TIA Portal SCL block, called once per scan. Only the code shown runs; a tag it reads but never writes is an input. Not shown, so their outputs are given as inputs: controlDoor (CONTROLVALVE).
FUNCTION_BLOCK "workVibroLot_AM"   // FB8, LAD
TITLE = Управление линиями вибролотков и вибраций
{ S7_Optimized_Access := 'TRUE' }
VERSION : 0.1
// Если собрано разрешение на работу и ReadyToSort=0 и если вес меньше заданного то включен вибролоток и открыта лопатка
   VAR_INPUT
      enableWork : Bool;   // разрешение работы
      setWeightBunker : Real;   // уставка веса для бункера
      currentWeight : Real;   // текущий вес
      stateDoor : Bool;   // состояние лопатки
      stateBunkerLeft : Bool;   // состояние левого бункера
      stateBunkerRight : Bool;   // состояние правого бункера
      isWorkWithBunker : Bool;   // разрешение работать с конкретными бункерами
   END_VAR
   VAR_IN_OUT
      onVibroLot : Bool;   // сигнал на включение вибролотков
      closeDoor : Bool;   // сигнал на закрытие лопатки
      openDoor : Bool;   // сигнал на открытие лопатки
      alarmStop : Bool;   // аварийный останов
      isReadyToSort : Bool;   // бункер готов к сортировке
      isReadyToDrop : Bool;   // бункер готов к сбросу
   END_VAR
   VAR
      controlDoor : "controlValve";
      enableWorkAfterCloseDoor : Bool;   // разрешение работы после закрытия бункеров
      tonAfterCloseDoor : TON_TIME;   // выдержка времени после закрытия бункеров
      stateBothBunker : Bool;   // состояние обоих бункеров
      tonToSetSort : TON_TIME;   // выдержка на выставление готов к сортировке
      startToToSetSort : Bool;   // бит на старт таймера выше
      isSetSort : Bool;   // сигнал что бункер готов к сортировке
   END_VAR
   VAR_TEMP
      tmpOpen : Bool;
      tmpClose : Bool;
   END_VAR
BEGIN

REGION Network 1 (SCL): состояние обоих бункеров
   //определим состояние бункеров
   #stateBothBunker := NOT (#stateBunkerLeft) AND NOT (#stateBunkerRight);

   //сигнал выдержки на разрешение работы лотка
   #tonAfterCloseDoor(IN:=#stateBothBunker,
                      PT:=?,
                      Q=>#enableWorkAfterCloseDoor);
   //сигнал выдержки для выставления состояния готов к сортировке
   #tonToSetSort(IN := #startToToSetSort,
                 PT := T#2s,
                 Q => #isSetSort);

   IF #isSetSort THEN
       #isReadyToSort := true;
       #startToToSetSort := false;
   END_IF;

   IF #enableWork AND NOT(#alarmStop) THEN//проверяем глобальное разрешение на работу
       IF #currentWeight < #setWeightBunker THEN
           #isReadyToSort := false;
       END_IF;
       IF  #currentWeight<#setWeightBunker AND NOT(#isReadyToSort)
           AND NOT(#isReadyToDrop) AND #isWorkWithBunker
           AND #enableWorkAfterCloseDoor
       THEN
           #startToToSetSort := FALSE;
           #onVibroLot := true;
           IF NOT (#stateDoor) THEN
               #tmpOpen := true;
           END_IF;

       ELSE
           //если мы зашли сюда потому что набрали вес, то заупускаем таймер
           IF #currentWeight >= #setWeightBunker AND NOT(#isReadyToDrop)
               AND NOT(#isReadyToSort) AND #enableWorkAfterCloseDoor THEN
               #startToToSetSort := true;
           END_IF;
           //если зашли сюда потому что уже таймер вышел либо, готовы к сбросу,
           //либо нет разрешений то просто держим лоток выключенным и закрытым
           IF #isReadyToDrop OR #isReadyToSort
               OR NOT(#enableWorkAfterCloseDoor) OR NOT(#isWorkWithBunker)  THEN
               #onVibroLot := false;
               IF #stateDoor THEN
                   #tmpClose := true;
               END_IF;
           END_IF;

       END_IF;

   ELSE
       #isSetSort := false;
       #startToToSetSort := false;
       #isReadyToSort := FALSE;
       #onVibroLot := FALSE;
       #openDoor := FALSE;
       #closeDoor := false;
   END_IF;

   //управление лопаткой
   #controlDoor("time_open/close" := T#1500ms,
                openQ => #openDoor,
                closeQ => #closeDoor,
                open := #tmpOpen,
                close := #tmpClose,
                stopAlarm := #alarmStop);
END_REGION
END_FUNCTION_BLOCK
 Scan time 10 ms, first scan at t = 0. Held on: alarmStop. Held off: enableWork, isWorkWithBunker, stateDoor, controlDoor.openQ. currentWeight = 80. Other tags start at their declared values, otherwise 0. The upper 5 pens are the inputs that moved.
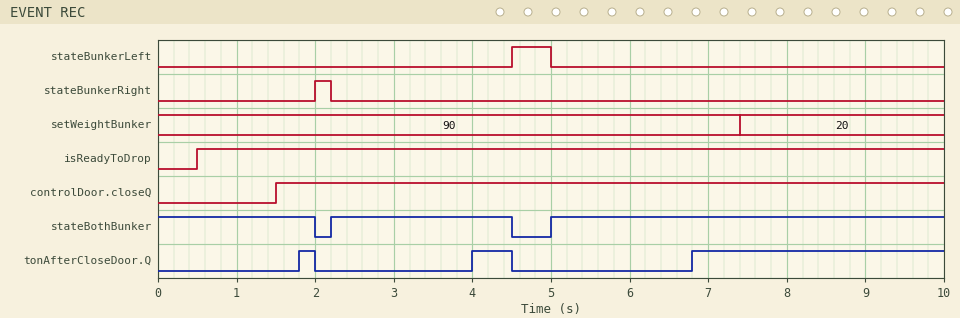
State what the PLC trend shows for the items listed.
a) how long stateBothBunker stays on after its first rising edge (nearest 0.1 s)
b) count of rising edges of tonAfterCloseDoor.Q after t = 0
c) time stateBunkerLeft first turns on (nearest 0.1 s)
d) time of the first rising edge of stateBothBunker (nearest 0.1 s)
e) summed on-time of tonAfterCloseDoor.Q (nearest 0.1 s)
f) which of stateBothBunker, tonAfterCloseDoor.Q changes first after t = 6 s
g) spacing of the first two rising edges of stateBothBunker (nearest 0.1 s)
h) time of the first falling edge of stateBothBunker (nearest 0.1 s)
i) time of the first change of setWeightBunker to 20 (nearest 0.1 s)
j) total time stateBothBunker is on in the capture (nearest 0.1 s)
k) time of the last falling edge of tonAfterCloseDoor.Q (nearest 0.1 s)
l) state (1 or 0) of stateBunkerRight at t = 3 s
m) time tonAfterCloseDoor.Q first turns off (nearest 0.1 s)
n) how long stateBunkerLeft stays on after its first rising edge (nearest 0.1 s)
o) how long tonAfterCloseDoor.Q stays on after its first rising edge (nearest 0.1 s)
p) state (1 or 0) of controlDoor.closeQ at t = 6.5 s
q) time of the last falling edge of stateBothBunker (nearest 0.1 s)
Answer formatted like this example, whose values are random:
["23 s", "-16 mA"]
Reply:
["2.3 s", "3", "4.5 s", "2.2 s", "3.9 s", "tonAfterCloseDoor.Q", "2.8 s", "2.0 s", "7.4 s", "9.3 s", "4.5 s", "0", "2.0 s", "0.5 s", "0.2 s", "1", "4.5 s"]
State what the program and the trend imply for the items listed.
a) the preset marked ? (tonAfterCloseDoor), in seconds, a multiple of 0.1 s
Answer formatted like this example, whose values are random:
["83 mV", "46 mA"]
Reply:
["1.8 s"]
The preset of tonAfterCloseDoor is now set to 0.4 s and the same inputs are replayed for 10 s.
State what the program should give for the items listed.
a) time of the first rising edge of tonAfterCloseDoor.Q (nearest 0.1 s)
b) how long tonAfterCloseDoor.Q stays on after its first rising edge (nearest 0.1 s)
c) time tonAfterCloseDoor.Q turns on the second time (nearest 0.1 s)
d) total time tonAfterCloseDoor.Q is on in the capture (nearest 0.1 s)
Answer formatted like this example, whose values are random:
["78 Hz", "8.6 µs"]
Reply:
["0.4 s", "1.6 s", "2.6 s", "8.1 s"]
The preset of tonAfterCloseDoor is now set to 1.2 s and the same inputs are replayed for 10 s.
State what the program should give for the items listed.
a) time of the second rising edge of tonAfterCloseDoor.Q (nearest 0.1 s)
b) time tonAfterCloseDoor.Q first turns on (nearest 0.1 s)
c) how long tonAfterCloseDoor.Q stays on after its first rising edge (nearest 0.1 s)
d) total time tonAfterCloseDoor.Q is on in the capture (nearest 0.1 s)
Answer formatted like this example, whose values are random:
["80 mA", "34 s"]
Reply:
["3.4 s", "1.2 s", "0.8 s", "5.7 s"]
